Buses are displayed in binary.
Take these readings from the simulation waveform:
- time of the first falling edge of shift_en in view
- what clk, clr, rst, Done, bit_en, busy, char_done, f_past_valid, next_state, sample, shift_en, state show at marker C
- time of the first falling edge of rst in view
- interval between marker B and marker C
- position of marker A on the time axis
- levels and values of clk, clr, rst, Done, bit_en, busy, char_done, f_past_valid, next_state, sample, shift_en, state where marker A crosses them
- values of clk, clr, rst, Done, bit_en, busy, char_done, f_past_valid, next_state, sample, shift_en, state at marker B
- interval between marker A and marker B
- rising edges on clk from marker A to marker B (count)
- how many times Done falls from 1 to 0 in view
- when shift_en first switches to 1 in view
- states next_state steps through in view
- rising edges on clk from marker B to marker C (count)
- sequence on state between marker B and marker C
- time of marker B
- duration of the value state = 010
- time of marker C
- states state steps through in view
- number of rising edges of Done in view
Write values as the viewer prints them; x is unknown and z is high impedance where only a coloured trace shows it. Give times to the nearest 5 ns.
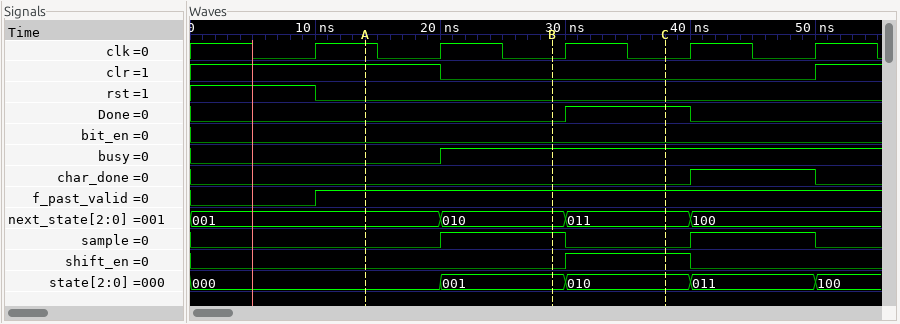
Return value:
40 ns
clk=0, clr=0, rst=0, Done=1, bit_en=0, busy=1, char_done=0, f_past_valid=1, next_state=011, sample=0, shift_en=1, state=010
10 ns
10 ns
15 ns
clk=1, clr=1, rst=0, Done=0, bit_en=0, busy=0, char_done=0, f_past_valid=1, next_state=001, sample=0, shift_en=0, state=000
clk=0, clr=0, rst=0, Done=0, bit_en=0, busy=1, char_done=0, f_past_valid=1, next_state=010, sample=1, shift_en=0, state=001
15 ns
1
1
30 ns
001, 010, 011, 100
1
001, 010
30 ns
10 ns
40 ns
000, 001, 010, 011, 100
1
